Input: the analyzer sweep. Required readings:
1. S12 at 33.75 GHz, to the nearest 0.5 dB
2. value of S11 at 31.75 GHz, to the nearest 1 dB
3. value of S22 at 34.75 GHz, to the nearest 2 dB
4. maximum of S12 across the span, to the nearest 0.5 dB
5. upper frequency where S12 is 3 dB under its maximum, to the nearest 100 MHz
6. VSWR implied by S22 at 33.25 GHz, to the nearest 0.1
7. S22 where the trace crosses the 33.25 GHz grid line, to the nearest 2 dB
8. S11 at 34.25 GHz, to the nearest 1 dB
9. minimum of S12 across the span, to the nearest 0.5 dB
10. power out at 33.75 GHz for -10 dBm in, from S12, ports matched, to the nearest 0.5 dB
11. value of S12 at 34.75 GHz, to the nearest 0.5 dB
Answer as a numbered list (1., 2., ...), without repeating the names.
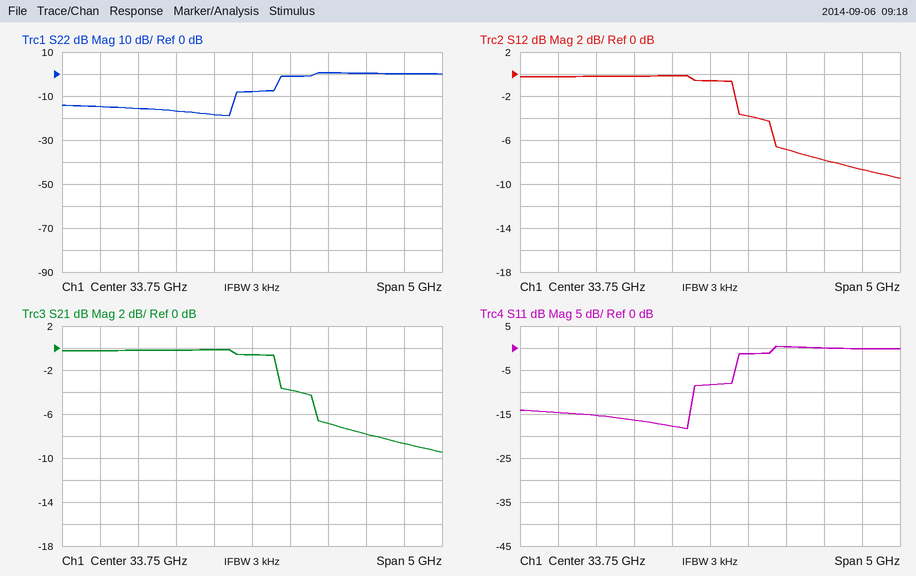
1. -0.5 dB
2. -15 dB
3. 0 dB
4. 0.0 dB
5. 34.1 GHz
6. 1.3
7. -18 dB
8. -1 dB
9. -9.5 dB
10. -10.5 dBm
11. -7.0 dB
